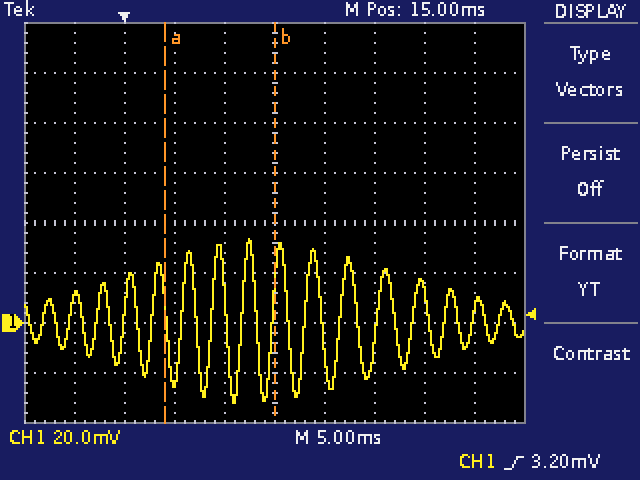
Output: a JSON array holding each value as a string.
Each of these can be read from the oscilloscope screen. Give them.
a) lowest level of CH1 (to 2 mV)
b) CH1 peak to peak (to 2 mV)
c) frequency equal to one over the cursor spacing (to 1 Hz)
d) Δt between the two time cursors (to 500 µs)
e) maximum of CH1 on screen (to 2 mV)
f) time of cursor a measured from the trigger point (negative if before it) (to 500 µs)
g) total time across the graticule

["-32 mV", "66 mV", "91 Hz", "11.0 ms", "34 mV", "+4.0 ms", "50 ms"]
